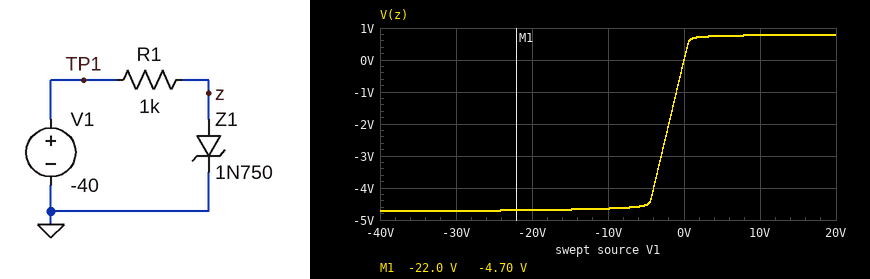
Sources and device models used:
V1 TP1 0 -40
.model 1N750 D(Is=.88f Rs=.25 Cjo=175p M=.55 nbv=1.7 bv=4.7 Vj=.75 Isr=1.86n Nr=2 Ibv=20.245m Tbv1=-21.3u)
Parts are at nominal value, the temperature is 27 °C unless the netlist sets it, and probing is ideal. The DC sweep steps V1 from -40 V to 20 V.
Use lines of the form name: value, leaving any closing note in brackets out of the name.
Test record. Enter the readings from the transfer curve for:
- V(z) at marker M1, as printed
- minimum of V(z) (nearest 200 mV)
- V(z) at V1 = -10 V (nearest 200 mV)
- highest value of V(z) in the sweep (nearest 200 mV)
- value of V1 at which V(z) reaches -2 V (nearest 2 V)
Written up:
V(z) at marker M1, as printed: -4.70 V
minimum of V(z): -4.8 V
V(z) at V1 = -10 V: -4.6 V
highest value of V(z) in the sweep: 800 mV
value of V1 at which V(z) reaches -2 V: -2 V
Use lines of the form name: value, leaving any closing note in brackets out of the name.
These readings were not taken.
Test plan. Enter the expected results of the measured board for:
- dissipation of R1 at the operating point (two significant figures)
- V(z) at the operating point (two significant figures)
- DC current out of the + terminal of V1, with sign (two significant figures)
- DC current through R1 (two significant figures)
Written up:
dissipation of R1 at the operating point: 1.2 W
V(z) at the operating point: -4.7 V
DC current out of the + terminal of V1, with sign: -35 mA
DC current through R1: 35 mA
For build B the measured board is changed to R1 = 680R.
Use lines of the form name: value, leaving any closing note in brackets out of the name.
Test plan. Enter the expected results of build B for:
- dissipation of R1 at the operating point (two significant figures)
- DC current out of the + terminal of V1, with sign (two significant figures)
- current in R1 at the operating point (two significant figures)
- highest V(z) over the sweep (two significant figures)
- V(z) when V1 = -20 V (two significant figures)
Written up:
dissipation of R1 at the operating point: 1.8 W
DC current out of the + terminal of V1, with sign: -52 mA
current in R1 at the operating point: 52 mA
highest V(z) over the sweep: 810 mV
V(z) when V1 = -20 V: -4.7 V
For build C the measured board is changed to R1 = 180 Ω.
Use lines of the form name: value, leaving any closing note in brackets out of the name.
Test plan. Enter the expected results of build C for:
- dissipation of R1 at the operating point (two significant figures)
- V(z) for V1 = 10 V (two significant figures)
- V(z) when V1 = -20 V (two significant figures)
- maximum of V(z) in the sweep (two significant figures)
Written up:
dissipation of R1 at the operating point: 6.9 W
V(z) for V1 = 10 V: 830 mV
V(z) when V1 = -20 V: -4.8 V
maximum of V(z) in the sweep: 860 mV
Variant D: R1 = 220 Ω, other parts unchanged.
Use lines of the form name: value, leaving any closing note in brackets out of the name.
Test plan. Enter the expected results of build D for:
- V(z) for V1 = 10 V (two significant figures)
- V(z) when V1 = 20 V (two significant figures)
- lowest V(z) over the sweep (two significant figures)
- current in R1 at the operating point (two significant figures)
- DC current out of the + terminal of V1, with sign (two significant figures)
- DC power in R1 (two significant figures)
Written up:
V(z) for V1 = 10 V: 820 mV
V(z) when V1 = 20 V: 850 mV
lowest V(z) over the sweep: -4.8 V
current in R1 at the operating point: 160 mA
DC current out of the + terminal of V1, with sign: -160 mA
DC power in R1: 5.6 W
